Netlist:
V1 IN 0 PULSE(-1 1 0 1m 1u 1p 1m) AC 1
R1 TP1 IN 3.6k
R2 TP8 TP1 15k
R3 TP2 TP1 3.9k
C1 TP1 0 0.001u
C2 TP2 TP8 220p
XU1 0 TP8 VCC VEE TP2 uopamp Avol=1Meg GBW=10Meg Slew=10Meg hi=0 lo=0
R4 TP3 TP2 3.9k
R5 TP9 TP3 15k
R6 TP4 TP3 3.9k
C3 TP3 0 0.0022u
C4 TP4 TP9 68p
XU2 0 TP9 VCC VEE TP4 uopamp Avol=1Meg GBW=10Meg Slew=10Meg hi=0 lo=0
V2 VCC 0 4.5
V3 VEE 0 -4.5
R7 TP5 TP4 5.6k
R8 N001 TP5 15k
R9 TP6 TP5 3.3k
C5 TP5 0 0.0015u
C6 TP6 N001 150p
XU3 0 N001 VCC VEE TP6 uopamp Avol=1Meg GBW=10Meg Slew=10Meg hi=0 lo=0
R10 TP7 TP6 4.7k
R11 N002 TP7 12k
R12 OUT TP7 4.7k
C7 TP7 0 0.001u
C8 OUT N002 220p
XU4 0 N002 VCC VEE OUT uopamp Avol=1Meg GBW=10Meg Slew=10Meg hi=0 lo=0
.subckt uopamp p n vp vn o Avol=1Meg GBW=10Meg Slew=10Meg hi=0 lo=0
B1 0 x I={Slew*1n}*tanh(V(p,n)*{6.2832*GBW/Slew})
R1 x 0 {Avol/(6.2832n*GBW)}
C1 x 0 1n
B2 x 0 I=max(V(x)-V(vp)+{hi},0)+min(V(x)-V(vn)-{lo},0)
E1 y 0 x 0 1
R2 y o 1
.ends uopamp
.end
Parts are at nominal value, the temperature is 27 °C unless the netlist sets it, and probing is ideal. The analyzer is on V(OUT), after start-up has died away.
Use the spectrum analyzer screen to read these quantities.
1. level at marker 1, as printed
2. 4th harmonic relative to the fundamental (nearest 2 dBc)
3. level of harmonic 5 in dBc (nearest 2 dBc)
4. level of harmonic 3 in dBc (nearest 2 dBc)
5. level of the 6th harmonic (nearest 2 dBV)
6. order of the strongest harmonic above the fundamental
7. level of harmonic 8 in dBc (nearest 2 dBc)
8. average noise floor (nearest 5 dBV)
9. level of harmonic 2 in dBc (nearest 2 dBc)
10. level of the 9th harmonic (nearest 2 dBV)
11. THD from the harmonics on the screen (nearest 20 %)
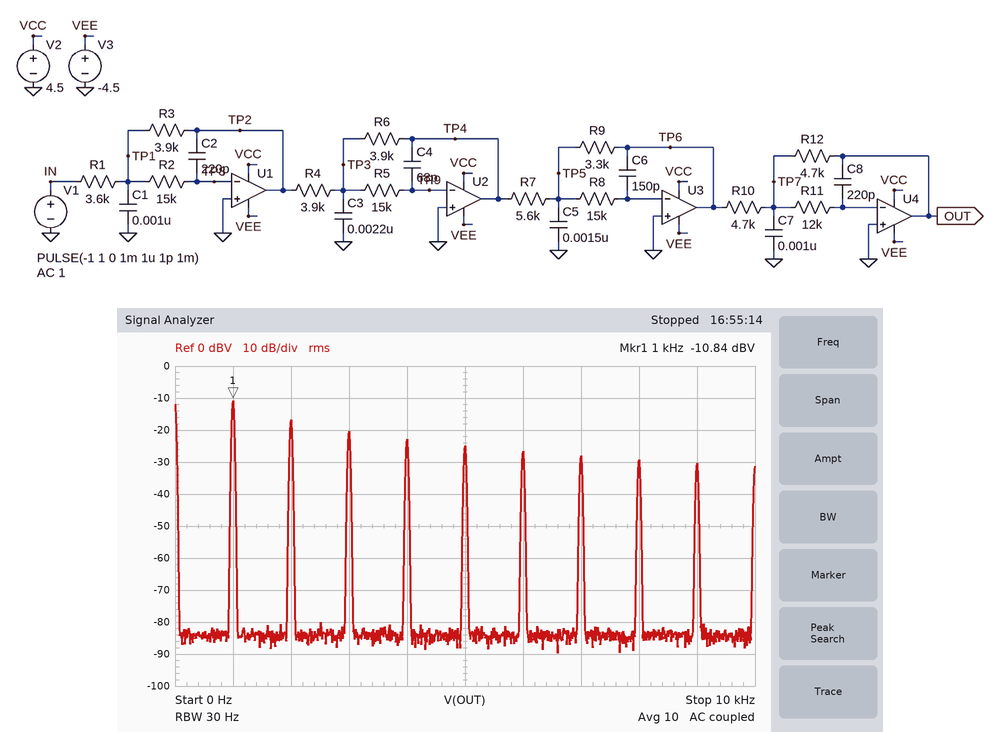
-10.84 dBV
-12 dBc
-14 dBc
-10 dBc
-26 dBV
2
-18 dBc
-85 dBV
-6 dBc
-30 dBV
80 %
